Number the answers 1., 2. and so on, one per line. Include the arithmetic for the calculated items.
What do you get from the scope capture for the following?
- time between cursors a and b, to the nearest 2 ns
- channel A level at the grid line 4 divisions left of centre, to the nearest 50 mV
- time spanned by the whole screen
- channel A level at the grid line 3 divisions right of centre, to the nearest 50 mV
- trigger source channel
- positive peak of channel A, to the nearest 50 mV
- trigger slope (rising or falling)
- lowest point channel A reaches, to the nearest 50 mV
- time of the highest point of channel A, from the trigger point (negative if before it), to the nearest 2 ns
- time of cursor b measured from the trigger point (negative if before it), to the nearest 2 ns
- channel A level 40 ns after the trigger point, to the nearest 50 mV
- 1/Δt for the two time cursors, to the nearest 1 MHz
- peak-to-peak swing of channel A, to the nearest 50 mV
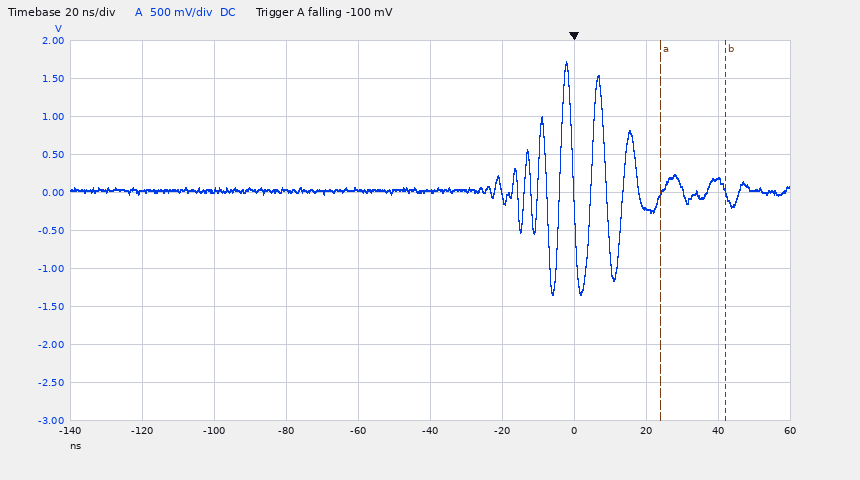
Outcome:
1. 18 ns
2. 0 mV
3. 200 ns
4. -200 mV
5. channel A
6. 1.70 V
7. falling
8. -1.35 V
9. -2 ns
10. +42 ns
11. 150 mV
12. 1 / 18 ns ≈ 56 MHz
13. 1.70 V − (-1.35 V) = 3.05 V
